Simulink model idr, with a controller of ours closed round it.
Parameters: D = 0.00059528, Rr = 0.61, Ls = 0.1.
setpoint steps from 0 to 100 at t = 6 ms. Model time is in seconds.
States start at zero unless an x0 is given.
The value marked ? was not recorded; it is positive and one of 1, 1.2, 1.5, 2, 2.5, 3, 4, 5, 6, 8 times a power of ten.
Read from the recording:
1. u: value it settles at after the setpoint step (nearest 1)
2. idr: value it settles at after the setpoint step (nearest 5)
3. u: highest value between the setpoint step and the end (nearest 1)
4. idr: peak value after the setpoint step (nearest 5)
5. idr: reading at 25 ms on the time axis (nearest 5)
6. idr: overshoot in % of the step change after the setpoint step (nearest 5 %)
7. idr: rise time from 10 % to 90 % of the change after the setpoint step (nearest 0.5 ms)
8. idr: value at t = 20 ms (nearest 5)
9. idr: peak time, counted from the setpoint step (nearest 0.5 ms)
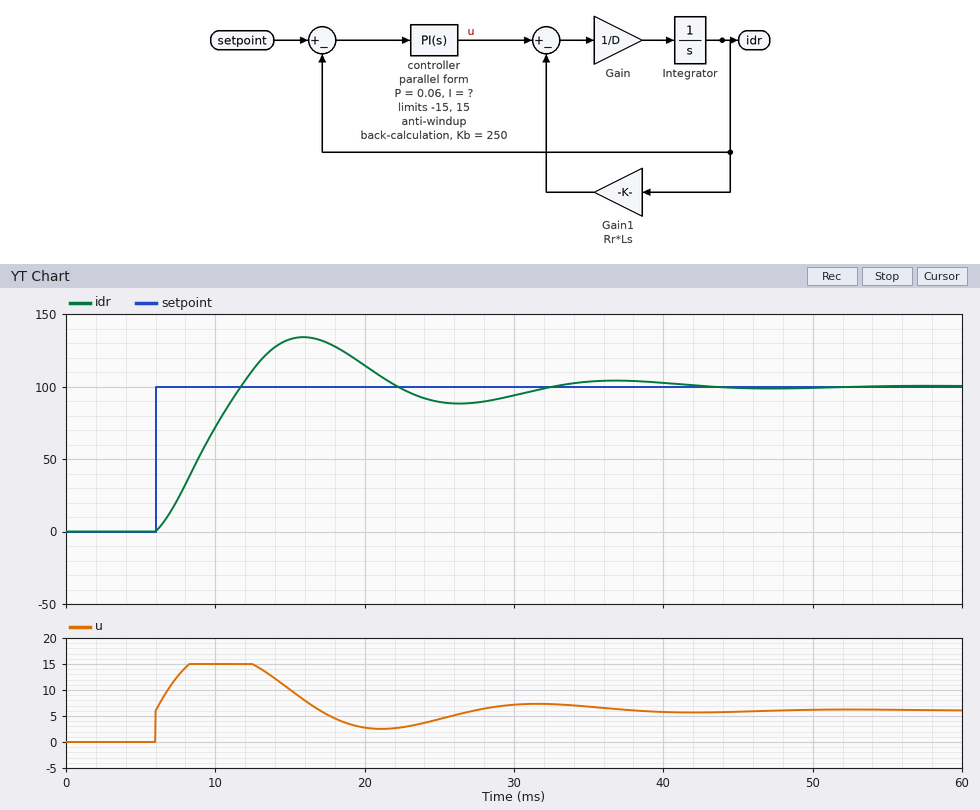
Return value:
6
100
15
135
90
35 %
4.5 ms
115
10.0 ms
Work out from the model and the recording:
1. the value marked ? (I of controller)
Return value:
60
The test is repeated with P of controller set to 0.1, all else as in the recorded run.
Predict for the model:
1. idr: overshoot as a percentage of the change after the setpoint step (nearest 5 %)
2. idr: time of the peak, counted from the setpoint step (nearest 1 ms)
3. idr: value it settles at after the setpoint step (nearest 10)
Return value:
25 %
9 ms
100
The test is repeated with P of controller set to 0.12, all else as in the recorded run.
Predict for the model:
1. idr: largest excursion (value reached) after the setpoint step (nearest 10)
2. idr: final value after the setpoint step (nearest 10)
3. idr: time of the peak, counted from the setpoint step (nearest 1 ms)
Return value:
120
100
9 ms
